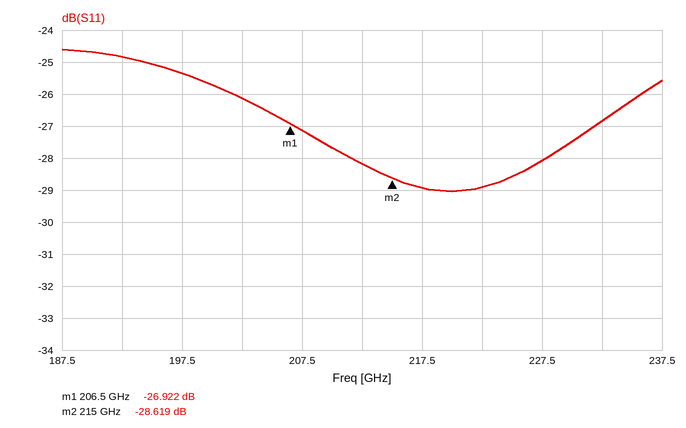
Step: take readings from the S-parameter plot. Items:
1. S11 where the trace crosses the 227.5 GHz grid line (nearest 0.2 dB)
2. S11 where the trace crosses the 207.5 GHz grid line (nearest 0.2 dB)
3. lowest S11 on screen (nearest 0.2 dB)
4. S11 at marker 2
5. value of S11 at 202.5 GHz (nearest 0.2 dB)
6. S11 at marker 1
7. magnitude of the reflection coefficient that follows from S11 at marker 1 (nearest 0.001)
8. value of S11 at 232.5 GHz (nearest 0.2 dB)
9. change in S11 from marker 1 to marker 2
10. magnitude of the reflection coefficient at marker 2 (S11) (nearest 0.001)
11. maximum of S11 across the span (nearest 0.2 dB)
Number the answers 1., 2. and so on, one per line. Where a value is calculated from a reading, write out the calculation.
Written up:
1. -28.0 dB
2. -27.2 dB
3. -29.0 dB
4. -28.619 dB
5. -26.2 dB
6. -26.922 dB
7. 10^(-26.922/20) ≈ 0.045
8. -26.8 dB
9. -28.619 − (-26.922) = -1.697 dB
10. 10^(-28.619/20) ≈ 0.037
11. -24.6 dB
